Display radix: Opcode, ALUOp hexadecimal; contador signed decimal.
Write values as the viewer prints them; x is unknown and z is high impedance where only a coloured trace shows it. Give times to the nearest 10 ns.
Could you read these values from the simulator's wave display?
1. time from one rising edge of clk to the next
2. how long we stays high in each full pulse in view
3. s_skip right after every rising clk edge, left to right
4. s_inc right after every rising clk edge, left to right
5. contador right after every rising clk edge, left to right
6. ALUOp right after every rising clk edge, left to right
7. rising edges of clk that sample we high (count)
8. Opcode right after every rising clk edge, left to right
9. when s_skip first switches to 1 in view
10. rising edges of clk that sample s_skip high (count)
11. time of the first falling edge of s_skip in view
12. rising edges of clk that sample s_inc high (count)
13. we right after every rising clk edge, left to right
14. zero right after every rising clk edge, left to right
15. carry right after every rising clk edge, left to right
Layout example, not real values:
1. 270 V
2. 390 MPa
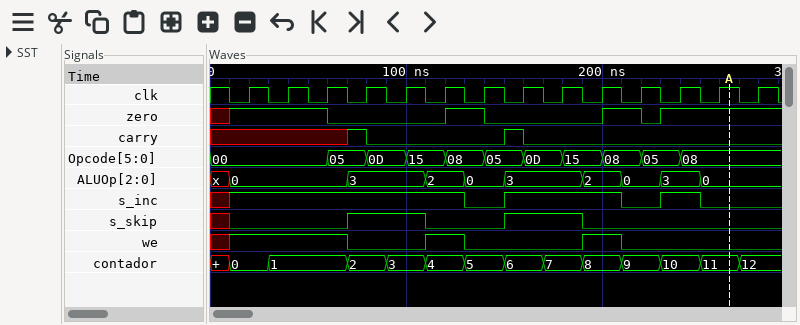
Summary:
1. 20 ns
2. 20 ns, 20 ns
3. 0 0 0 1 1 0 0 1 1 0 0 0 0 0
4. 1 1 1 1 1 1 0 1 1 1 0 1 0 0
5. 0, 1, 1, 2, 3, 4, 5, 6, 7, 8, 9, 10, 11, 12
6. 0, 0, 0, 3, 3, 2, 0, 3, 3, 2, 0, 3, 0, 0
7. 5
8. 00, 00, 05, 0D, 15, 08, 05, 0D, 15, 08, 05, 08, 08, 08
9. 70 ns
10. 4
11. 110 ns
12. 10
13. 1 1 1 0 0 1 0 0 0 1 0 0 0 0
14. 1 1 0 0 0 1 0 0 0 1 0 1 1 1
15. x x x 0 0 0 0 0 0 0 0 0 0 0
